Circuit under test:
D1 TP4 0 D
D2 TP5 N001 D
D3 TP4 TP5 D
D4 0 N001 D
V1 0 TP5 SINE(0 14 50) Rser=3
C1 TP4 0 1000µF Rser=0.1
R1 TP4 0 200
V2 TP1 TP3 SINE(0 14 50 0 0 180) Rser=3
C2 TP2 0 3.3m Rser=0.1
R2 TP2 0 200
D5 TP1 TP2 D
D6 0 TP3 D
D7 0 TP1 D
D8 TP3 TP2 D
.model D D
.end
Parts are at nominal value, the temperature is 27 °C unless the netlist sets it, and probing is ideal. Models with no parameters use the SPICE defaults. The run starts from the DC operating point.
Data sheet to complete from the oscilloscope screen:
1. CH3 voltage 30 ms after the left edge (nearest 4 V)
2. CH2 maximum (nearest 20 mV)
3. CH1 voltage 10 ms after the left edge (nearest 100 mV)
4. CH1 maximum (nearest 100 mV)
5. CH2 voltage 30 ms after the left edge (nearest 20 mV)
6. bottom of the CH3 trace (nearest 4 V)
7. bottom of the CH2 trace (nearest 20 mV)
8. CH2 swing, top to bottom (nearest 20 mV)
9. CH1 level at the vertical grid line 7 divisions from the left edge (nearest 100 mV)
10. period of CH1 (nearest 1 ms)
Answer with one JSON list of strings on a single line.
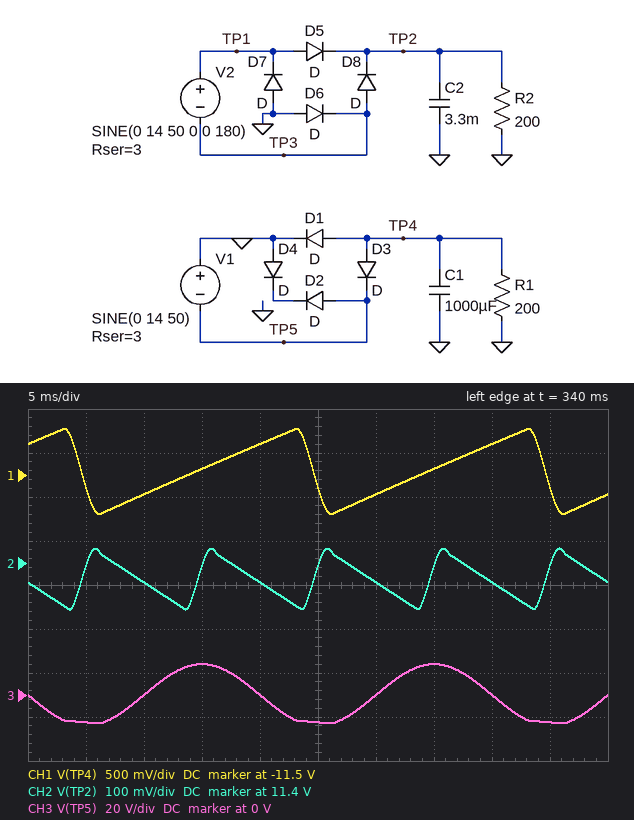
["0 V", "11.44 V", "-11.7 V", "-11.0 V", "11.36 V", "-12 V", "11.30 V", "140 mV", "-11.4 V", "20 ms"]
